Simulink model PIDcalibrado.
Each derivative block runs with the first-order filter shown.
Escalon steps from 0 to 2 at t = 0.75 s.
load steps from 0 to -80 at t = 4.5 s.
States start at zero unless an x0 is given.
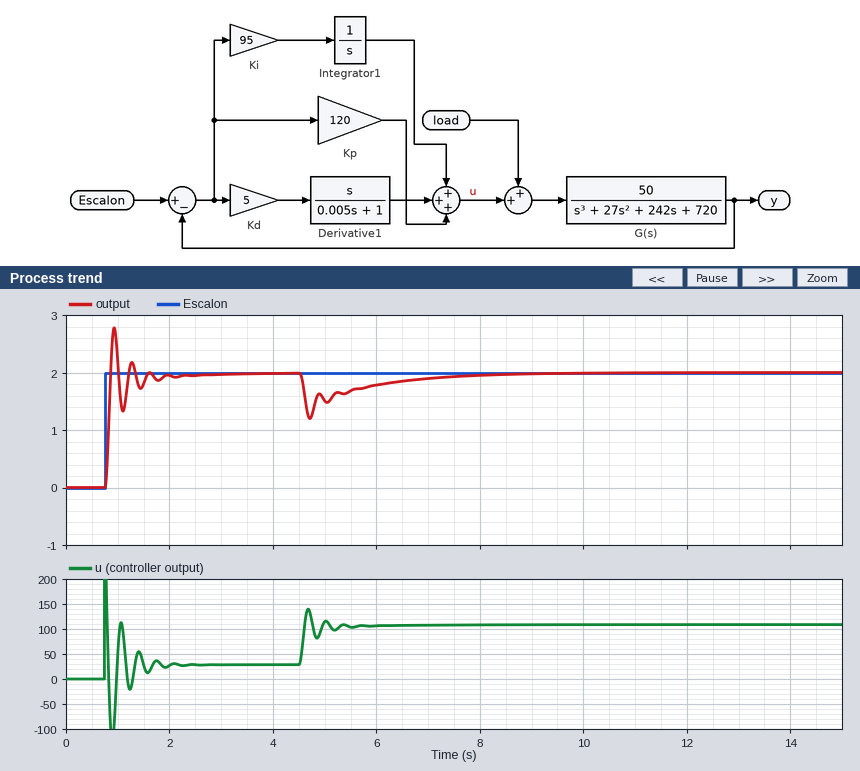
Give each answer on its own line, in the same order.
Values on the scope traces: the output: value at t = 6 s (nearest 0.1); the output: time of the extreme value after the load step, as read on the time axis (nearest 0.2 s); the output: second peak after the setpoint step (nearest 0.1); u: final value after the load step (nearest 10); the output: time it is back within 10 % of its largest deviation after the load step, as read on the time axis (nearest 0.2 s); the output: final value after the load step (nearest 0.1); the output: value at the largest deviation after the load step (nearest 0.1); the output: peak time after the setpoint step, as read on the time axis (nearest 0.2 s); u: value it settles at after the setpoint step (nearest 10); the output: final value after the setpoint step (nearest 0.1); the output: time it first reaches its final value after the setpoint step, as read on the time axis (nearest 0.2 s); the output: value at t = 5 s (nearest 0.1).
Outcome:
1.8
4.8 s
2.2
110
7.4 s
2.0
1.2
1.0 s
30
2.0
0.8 s
1.5
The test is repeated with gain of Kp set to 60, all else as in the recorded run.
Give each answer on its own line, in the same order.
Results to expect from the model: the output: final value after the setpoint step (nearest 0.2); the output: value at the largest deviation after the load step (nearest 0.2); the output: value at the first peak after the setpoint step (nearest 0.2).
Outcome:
2.0
1.0
2.2
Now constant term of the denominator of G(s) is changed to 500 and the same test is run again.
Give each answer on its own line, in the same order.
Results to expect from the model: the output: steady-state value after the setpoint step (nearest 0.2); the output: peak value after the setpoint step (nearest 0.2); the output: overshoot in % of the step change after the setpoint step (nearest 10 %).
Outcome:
2.0
2.8
40 %
